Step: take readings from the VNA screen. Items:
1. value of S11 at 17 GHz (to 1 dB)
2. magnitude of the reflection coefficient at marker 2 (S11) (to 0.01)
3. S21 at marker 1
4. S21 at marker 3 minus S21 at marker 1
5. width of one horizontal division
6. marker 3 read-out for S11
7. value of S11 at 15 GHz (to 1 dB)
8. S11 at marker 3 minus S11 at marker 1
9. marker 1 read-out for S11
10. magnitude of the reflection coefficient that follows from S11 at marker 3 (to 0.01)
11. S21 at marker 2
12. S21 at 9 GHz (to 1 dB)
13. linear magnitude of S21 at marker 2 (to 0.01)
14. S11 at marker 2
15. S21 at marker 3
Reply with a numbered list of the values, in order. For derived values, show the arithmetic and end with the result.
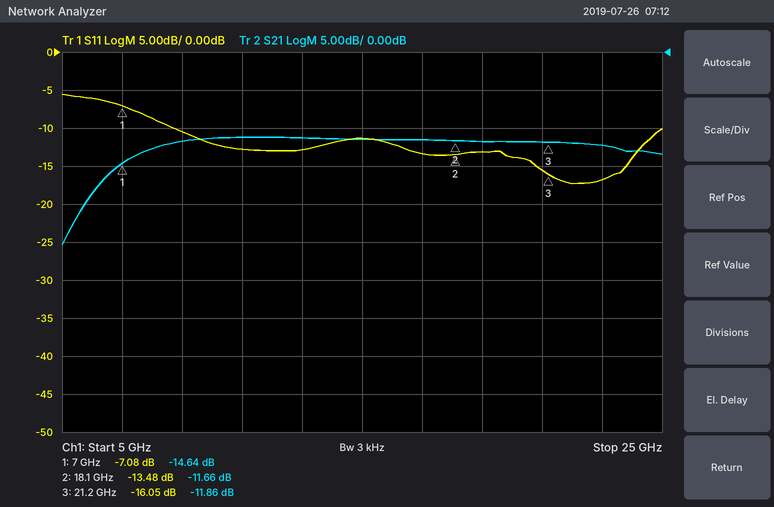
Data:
1. -13 dB
2. 10^(-13.48/20) ≈ 0.21
3. -14.64 dB
4. -11.86 − (-14.64) = 2.78 dB
5. 2 GHz
6. -16.05 dB
7. -11 dB
8. -16.05 − (-7.08) = -8.97 dB
9. -7.08 dB
10. 10^(-16.05/20) ≈ 0.16
11. -11.66 dB
12. -12 dB
13. 10^(-11.66/20) ≈ 0.26
14. -13.48 dB
15. -11.86 dB
